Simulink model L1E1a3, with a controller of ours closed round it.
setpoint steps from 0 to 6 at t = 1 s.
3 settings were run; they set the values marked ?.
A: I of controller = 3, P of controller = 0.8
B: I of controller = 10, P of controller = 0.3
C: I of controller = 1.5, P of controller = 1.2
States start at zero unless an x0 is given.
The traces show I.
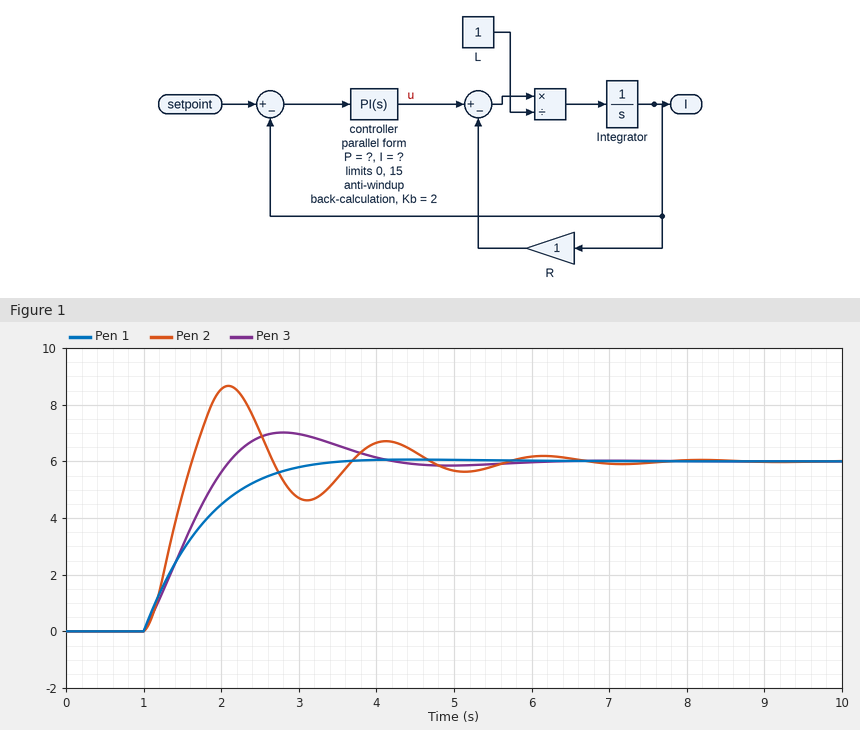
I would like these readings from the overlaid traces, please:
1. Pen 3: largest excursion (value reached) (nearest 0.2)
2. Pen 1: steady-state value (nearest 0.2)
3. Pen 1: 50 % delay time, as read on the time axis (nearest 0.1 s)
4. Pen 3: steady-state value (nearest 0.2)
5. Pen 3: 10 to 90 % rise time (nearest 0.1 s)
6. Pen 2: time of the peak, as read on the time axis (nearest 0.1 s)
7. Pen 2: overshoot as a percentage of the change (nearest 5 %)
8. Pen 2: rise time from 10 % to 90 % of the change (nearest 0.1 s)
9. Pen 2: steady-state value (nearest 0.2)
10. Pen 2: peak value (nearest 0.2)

7.0
6.0
1.5 s
6.0
0.8 s
2.1 s
45 %
0.4 s
6.0
8.6
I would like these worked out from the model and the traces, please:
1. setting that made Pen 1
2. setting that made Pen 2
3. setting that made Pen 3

C
B
A
